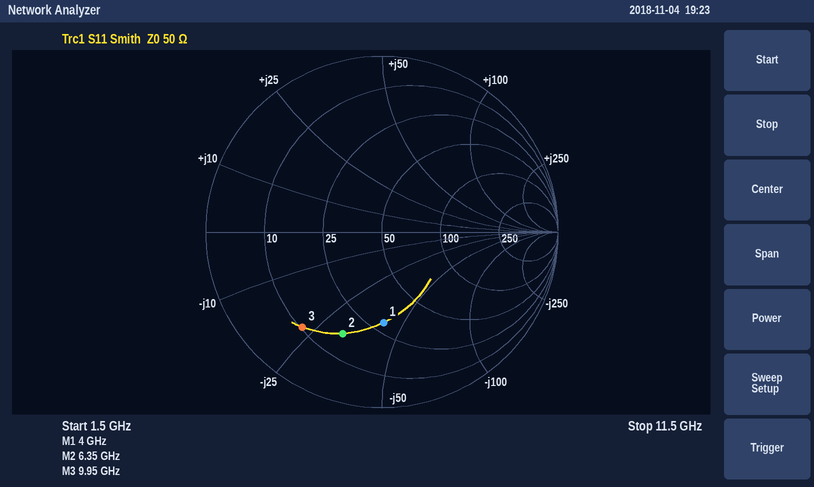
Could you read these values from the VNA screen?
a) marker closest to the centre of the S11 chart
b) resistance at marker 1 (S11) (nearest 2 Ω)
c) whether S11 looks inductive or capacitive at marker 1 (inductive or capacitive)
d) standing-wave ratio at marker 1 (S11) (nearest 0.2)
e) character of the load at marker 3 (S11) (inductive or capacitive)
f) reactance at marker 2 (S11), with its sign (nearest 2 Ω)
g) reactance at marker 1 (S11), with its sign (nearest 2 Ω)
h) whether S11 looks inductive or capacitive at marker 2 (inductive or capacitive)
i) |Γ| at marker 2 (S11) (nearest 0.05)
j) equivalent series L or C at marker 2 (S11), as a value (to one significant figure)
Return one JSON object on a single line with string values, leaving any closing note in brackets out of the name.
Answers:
{"marker closest to the centre of the S11 chart": "marker 1", "resistance at marker 1 (S11)": "30 Ω", "whether S11 looks inductive or capacitive at marker 1": "capacitive", "standing-wave ratio at marker 1 (S11)": "3.2", "character of the load at marker 3 (S11)": "capacitive", "reactance at marker 2 (S11), with its sign": "-32 Ω", "reactance at marker 1 (S11), with its sign": "-42 Ω", "whether S11 looks inductive or capacitive at marker 2": "capacitive", "|Γ| at marker 2 (S11)": "0.60", "equivalent series L or C at marker 2 (S11), as a value": "800 fF"}
